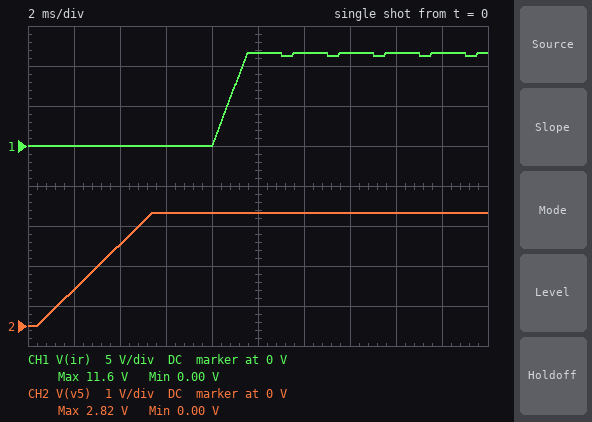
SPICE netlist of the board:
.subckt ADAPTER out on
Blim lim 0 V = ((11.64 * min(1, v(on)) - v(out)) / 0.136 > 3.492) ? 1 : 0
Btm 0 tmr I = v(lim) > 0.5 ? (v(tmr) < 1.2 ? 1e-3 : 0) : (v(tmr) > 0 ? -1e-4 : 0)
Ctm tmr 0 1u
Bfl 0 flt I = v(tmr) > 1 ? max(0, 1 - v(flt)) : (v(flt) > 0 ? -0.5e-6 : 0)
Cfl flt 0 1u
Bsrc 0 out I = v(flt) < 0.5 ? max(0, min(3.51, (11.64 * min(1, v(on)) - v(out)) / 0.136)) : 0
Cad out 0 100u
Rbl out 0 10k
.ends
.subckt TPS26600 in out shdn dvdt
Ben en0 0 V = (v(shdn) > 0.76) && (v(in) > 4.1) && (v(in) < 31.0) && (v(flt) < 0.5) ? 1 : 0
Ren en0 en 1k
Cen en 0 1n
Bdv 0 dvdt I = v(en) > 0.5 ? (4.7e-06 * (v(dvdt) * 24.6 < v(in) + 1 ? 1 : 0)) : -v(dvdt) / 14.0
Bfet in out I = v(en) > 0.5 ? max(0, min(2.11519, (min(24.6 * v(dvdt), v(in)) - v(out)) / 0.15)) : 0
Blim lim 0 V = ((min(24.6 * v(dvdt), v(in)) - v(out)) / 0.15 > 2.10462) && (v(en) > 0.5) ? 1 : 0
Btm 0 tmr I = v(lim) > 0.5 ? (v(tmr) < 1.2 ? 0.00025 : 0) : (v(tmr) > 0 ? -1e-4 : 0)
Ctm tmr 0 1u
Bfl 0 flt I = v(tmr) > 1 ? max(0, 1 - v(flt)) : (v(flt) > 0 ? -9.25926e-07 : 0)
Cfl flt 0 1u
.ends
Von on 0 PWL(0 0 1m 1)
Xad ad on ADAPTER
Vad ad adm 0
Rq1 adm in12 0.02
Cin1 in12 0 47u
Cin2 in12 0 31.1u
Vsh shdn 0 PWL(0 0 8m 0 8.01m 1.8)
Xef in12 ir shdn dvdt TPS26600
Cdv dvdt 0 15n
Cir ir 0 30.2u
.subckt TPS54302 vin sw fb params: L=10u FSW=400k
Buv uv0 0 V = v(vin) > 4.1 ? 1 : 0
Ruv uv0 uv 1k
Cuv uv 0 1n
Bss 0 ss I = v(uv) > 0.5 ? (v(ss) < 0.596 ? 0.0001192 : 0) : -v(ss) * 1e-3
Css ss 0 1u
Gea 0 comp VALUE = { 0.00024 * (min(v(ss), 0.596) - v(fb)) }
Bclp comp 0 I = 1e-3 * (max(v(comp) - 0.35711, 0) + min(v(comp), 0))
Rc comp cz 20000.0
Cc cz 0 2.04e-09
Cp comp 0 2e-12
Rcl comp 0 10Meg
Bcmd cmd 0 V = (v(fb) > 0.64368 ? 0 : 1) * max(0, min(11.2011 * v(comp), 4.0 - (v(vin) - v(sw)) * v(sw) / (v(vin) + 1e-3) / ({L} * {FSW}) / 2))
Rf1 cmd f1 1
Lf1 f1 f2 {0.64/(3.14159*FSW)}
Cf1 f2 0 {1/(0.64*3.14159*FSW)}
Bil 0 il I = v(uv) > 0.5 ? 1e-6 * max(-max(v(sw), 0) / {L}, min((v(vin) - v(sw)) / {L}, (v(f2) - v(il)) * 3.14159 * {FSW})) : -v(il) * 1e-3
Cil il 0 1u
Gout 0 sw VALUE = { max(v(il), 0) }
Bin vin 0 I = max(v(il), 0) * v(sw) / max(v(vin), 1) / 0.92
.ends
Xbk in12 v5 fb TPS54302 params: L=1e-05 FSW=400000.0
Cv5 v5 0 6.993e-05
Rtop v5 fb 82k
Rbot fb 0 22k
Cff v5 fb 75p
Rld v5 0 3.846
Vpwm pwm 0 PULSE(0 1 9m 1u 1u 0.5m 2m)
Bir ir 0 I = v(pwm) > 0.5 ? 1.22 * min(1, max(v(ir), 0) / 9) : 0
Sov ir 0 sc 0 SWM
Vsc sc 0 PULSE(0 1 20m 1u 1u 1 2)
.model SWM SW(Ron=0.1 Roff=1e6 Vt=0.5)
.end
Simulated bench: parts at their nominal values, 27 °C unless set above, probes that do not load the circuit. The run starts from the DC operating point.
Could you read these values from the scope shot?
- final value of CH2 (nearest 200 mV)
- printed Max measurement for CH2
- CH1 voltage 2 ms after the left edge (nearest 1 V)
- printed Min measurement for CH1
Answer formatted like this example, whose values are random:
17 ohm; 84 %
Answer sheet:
2.8 V; 2.82 V; 0 V; 0.00 V
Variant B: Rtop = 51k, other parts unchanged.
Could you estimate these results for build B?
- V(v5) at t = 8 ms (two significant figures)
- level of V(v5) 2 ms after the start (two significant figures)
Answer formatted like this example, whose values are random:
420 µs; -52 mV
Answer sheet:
2.0 V; 640 mV
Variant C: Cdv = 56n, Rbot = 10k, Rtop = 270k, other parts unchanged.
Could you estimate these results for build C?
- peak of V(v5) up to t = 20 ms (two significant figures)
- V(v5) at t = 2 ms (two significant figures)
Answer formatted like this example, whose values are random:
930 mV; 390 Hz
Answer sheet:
11 V; 5.3 V
